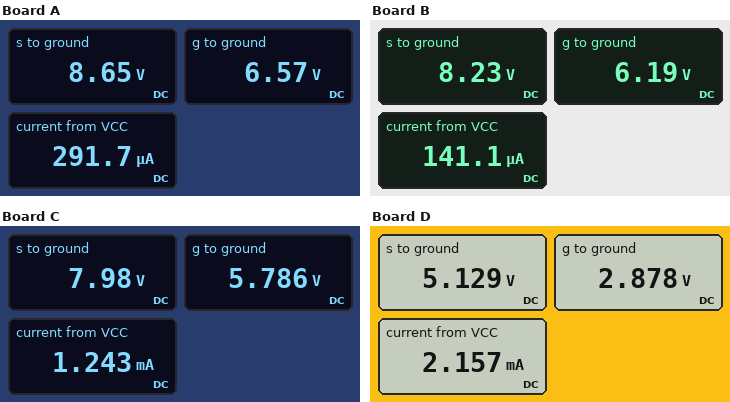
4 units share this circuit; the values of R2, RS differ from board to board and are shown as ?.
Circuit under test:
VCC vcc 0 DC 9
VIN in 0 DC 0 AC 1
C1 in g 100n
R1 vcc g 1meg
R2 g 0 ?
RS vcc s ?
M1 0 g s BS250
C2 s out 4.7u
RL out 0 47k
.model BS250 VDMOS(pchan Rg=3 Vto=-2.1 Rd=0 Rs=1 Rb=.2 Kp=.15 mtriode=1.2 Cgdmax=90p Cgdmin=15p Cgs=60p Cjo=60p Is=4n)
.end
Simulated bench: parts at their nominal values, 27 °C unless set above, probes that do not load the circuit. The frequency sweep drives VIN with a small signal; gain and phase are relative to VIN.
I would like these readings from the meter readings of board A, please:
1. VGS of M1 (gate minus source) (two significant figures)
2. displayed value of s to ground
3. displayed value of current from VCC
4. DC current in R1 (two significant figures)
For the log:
-2.1 V
8.65 V
291.7 µA
2.4 µA
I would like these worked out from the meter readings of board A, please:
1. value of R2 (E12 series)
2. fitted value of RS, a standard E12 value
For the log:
2.7 MΩ
1.2 kΩ
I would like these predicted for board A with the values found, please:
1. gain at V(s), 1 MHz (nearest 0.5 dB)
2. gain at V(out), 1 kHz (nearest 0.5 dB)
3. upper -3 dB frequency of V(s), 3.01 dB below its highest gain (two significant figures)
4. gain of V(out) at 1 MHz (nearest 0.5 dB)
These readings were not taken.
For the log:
-1.5 dB
-1.5 dB
1.3 GHz
-1.5 dB
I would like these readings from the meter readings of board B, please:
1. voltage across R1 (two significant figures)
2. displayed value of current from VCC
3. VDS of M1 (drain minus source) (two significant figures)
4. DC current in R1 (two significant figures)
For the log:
2.8 V
141.1 µA
-8.2 V
2.8 µA
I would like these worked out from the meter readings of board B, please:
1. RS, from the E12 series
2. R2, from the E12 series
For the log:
5.6 kΩ
2.2 MΩ
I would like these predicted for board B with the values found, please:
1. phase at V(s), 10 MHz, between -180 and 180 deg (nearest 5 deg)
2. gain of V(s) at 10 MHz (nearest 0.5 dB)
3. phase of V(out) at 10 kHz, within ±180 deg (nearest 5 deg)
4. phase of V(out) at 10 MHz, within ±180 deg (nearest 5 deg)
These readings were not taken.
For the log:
-5 deg
-2.0 dB
0 deg
-5 deg
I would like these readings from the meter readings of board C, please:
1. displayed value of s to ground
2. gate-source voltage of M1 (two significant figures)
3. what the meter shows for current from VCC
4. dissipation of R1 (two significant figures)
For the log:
7.98 V
-2.2 V
1.243 mA
10 µW
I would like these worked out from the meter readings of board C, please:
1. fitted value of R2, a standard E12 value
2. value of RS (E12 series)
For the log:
1.8 MΩ
820 Ω
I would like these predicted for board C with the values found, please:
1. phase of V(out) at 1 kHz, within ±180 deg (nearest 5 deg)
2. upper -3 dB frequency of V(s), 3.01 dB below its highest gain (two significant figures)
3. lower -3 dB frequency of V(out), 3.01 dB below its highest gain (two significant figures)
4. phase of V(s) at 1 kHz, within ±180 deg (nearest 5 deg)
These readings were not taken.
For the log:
0 deg
930 MHz
2.7 Hz
0 deg
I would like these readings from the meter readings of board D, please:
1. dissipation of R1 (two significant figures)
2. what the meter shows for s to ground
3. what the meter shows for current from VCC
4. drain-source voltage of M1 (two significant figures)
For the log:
37 µW
5.129 V
2.157 mA
-5.1 V
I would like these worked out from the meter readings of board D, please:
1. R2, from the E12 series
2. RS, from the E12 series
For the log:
470 kΩ
1.8 kΩ
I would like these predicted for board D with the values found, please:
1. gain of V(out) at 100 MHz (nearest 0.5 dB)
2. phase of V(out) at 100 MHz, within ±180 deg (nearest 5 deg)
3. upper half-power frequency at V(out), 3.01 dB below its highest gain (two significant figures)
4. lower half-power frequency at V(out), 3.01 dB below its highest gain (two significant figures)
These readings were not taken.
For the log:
-2.0 dB
-10 deg
480 MHz
5.1 Hz
